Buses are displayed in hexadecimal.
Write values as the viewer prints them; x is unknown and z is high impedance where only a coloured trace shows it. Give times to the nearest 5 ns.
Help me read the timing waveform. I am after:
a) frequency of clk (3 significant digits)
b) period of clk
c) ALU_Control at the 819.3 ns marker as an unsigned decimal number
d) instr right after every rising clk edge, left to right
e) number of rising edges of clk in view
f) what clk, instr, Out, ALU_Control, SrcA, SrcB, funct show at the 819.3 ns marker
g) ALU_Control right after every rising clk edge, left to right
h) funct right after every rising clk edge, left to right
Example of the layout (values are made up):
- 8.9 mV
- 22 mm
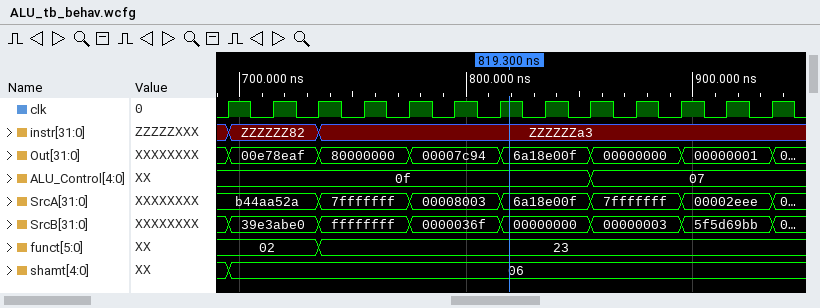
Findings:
- 50.0 MHz
- 20 ns
- 15
- ZZZZZZ82, ZZZZZZ82, ZZZZZZa3, ZZZZZZa3, ZZZZZZa3, ZZZZZZa3, ZZZZZZa3, ZZZZZZa3, ZZZZZZa3, ZZZZZZa3, ZZZZZZa3, ZZZZZZa3, ZZZZZZa3
- 13
- clk=1, instr=ZZZZZZa3, Out=6a18e00f, ALU_Control=0f, SrcA=6a18e00f, SrcB=00000000, funct=23
- 0f, 0f, 0f, 0f, 0f, 0f, 0f, 0f, 07, 07, 07, 07, 07
- 02, 02, 23, 23, 23, 23, 23, 23, 23, 23, 23, 23, 23
